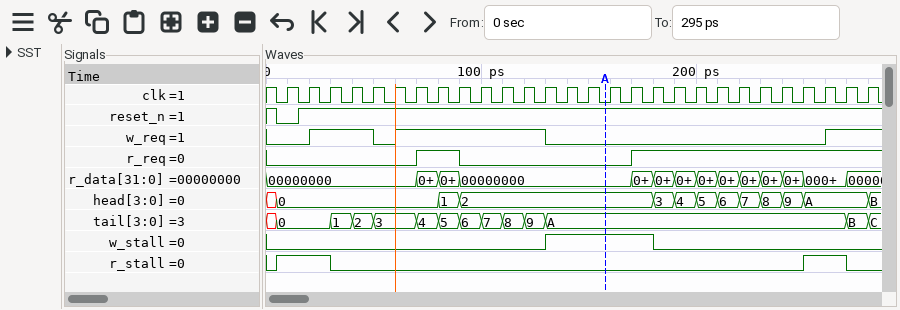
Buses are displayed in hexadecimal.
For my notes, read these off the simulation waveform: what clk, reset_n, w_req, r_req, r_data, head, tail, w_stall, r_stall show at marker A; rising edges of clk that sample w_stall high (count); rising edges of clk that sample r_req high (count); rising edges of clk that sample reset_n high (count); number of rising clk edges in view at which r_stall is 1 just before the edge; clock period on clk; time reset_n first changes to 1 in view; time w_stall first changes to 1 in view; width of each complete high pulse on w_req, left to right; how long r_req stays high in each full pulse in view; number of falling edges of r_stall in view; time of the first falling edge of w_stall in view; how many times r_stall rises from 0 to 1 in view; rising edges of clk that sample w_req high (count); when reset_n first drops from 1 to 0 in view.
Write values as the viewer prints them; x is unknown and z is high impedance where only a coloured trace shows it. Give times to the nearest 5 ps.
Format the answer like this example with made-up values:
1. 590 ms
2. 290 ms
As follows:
1. clk=0, reset_n=1, w_req=0, r_req=0, r_data=00000000, head=2, tail=A, w_stall=1, r_stall=0
2. 5
3. 13
4. 27
5. 5
6. 10 ps
7. 15 ps
8. 130 ps
9. 30 ps, 70 ps
10. 20 ps
11. 2
12. 180 ps
13. 2
14. 12
15. 5 ps
